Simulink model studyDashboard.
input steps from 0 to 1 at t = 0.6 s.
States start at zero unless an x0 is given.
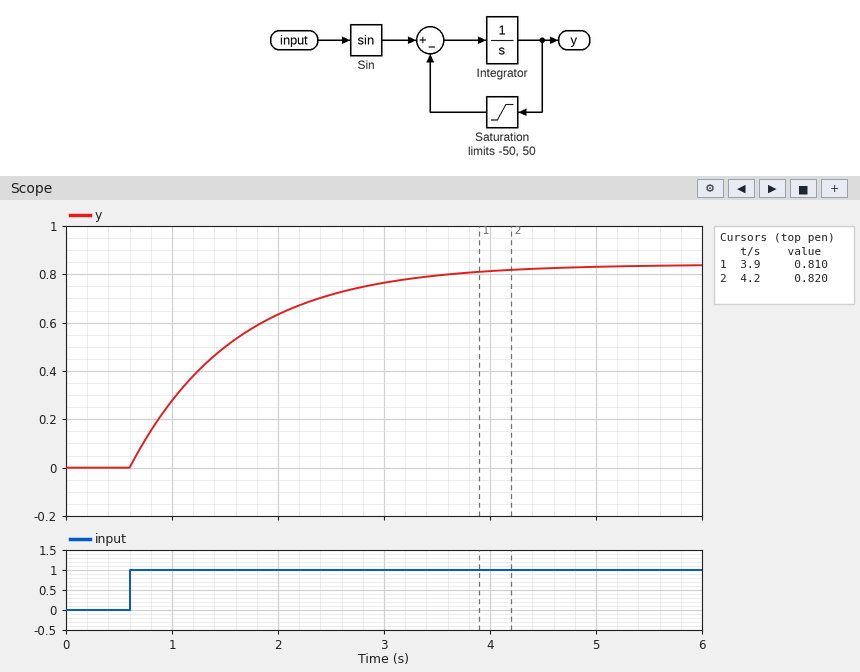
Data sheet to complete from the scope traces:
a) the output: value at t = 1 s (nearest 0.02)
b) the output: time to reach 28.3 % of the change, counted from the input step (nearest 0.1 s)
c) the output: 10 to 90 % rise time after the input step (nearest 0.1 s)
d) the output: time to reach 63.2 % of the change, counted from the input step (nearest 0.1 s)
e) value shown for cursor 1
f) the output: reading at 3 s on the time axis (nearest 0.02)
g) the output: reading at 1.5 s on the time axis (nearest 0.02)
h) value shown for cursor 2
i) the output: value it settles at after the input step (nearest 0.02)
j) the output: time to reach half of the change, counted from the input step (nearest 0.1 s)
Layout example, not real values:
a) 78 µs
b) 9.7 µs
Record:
a) 0.28
b) 0.3 s
c) 2.2 s
d) 1.0 s
e) 0.810
f) 0.76
g) 0.50
h) 0.820
i) 0.84
j) 0.7 s
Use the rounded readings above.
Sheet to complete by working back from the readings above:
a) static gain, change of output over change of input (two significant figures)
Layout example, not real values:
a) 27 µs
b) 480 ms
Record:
a) 0.84
